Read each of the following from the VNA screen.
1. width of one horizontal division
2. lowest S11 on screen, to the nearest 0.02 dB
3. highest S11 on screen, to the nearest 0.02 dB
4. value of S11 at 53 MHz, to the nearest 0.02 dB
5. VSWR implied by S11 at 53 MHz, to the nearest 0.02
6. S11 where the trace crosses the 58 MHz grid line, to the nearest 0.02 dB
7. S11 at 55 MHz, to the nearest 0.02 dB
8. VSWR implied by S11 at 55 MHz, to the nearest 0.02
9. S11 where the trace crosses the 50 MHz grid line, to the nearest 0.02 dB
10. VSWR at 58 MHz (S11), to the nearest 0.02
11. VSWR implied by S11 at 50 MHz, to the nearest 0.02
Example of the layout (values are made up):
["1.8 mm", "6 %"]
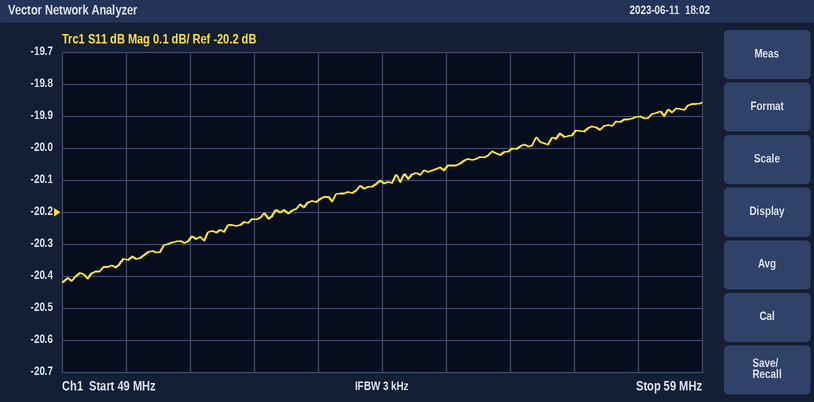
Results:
["1 MHz", "-20.42 dB", "-19.86 dB", "-20.16 dB", "1.22", "-19.90 dB", "-20.06 dB", "1.22", "-20.34 dB", "1.22", "1.22"]
